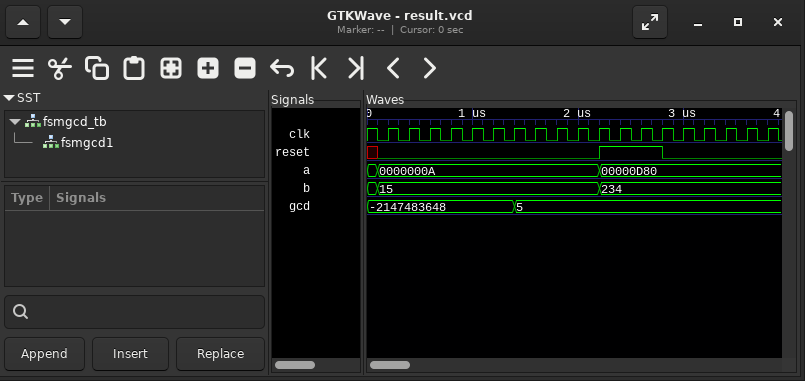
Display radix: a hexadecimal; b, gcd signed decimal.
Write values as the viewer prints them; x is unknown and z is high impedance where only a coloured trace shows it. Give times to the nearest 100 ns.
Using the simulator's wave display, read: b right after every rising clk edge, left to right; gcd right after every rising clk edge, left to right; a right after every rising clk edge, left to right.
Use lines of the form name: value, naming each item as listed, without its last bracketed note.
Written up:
b right after every rising clk edge, left to right: 15, 15, 15, 15, 15, 15, 15, 15, 15, 15, 234, 234, 234, 234, 234, 234, 234, 234, 234
gcd right after every rising clk edge, left to right: -2147483648, -2147483648, -2147483648, -2147483648, -2147483648, -2147483648, 5, 5, 5, 5, 5, 5, 5, 5, 5, 5, 5, 5, 5
a right after every rising clk edge, left to right: 0000000A, 0000000A, 0000000A, 0000000A, 0000000A, 0000000A, 0000000A, 0000000A, 0000000A, 0000000A, 00000D80, 00000D80, 00000D80, 00000D80, 00000D80, 00000D80, 00000D80, 00000D80, 00000D80
